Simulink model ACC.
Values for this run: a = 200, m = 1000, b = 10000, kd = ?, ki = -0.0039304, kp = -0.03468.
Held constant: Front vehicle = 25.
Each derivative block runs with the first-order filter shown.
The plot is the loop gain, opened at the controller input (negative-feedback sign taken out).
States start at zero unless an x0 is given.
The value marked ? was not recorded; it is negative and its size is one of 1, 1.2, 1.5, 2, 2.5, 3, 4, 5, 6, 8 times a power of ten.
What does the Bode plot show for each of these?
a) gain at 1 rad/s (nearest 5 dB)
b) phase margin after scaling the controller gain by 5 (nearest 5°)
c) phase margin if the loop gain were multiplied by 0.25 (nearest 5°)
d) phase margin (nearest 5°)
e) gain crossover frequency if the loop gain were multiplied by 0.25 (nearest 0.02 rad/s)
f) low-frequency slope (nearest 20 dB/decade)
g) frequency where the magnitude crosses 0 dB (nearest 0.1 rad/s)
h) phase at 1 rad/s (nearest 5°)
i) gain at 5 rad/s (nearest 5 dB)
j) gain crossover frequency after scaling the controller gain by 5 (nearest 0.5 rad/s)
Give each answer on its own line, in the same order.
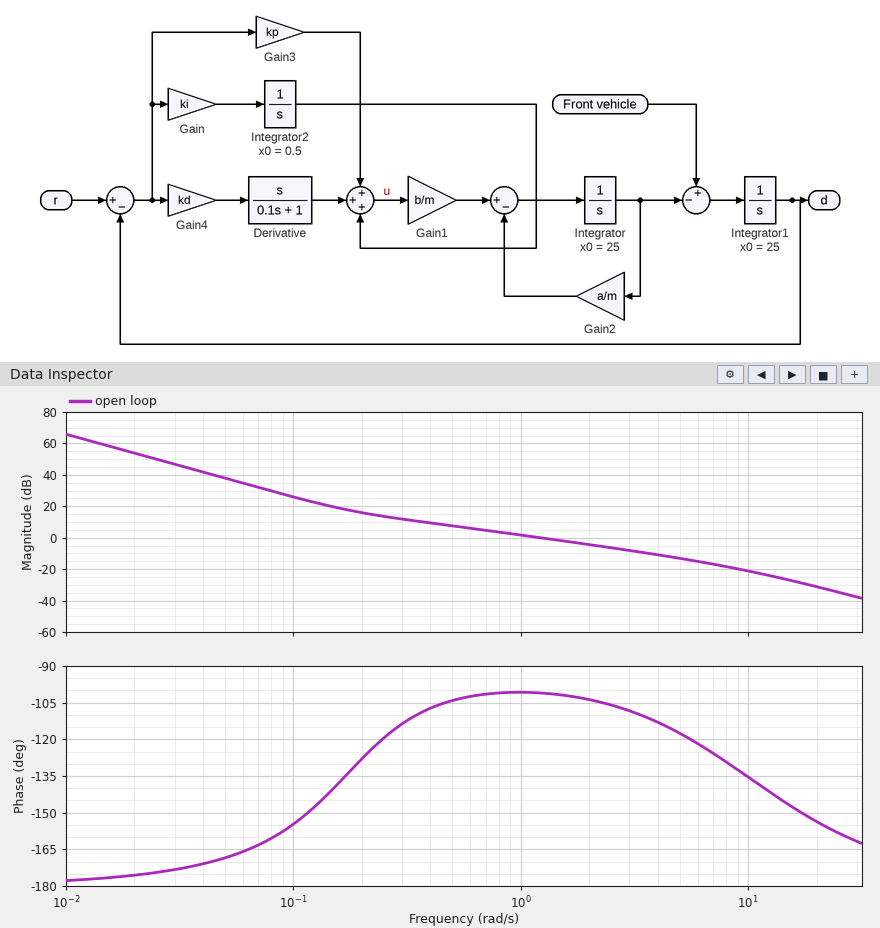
0 dB
60°
65°
80°
0.30 rad/s
-40 dB/decade
1.2 rad/s
-100°
-15 dB
5.5 rad/s
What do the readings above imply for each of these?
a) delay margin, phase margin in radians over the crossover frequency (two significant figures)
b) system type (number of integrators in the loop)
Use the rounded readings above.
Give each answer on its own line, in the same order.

1.2 s
2
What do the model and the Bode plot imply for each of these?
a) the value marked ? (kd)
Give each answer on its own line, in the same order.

-0.12
